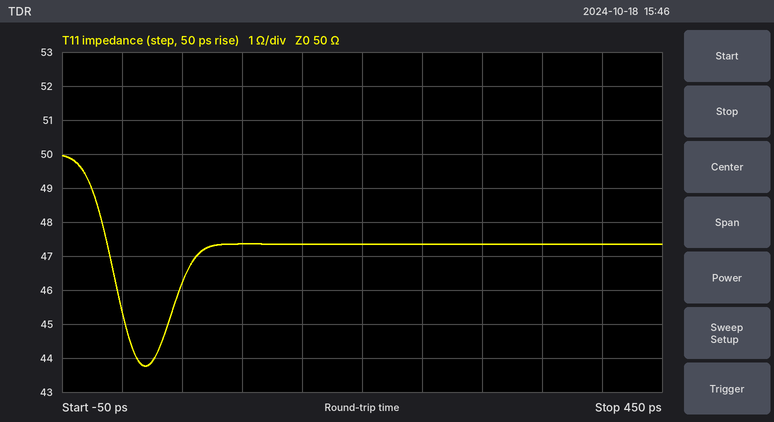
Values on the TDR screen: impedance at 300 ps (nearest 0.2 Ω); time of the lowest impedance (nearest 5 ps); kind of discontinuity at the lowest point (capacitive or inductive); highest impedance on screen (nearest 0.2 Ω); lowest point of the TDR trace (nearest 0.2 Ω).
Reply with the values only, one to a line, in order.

47.4 Ω
20 ps
capacitive
50.0 Ω
43.8 Ω
